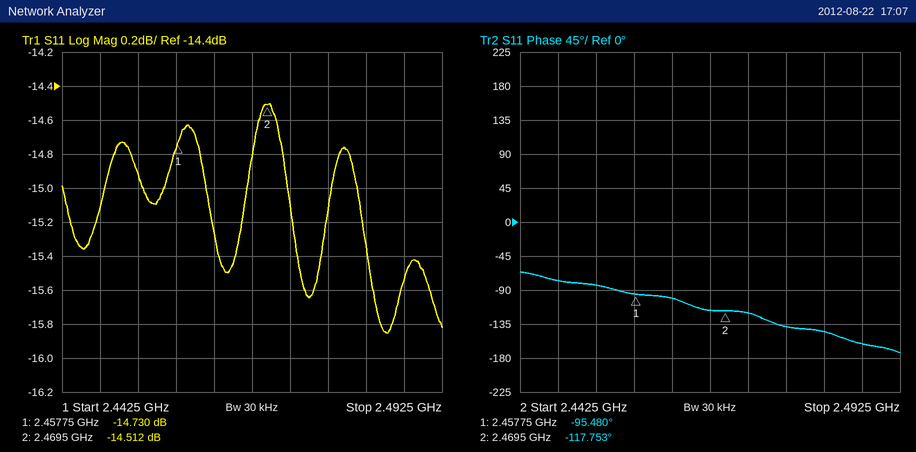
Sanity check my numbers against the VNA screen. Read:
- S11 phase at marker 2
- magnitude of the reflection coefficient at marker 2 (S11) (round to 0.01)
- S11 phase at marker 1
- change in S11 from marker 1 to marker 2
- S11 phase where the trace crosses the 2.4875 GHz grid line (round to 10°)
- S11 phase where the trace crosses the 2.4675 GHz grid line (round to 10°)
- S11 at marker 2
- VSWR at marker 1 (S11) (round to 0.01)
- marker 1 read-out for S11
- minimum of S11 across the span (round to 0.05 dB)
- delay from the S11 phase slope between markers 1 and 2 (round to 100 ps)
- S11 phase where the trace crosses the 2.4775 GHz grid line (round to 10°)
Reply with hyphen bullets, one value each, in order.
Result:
- -117.753°
- 0.19
- -95.480°
- 0.218 dB
- -160°
- -120°
- -14.512 dB
- 1.45
- -14.730 dB
- -15.85 dB
- 5.3 ns
- -140°
